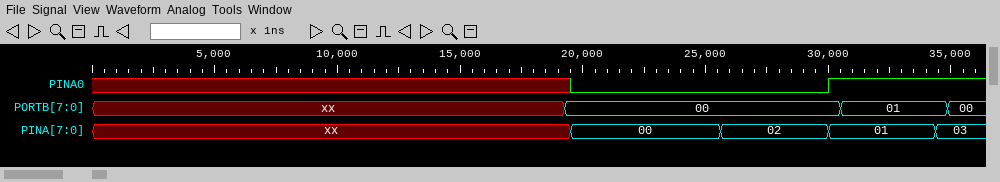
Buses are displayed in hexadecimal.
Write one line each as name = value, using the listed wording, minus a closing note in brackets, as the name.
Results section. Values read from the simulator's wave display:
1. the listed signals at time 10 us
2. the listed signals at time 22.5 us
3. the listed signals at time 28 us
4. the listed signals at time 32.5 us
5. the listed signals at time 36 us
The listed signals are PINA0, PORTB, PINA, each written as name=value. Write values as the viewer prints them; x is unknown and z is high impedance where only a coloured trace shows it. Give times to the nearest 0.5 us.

the listed signals at time 10 us = PINA0=x, PORTB=xx, PINA=xx
the listed signals at time 22.5 us = PINA0=0, PORTB=00, PINA=00
the listed signals at time 28 us = PINA0=0, PORTB=00, PINA=02
the listed signals at time 32.5 us = PINA0=1, PORTB=01, PINA=01
the listed signals at time 36 us = PINA0=1, PORTB=00, PINA=03
